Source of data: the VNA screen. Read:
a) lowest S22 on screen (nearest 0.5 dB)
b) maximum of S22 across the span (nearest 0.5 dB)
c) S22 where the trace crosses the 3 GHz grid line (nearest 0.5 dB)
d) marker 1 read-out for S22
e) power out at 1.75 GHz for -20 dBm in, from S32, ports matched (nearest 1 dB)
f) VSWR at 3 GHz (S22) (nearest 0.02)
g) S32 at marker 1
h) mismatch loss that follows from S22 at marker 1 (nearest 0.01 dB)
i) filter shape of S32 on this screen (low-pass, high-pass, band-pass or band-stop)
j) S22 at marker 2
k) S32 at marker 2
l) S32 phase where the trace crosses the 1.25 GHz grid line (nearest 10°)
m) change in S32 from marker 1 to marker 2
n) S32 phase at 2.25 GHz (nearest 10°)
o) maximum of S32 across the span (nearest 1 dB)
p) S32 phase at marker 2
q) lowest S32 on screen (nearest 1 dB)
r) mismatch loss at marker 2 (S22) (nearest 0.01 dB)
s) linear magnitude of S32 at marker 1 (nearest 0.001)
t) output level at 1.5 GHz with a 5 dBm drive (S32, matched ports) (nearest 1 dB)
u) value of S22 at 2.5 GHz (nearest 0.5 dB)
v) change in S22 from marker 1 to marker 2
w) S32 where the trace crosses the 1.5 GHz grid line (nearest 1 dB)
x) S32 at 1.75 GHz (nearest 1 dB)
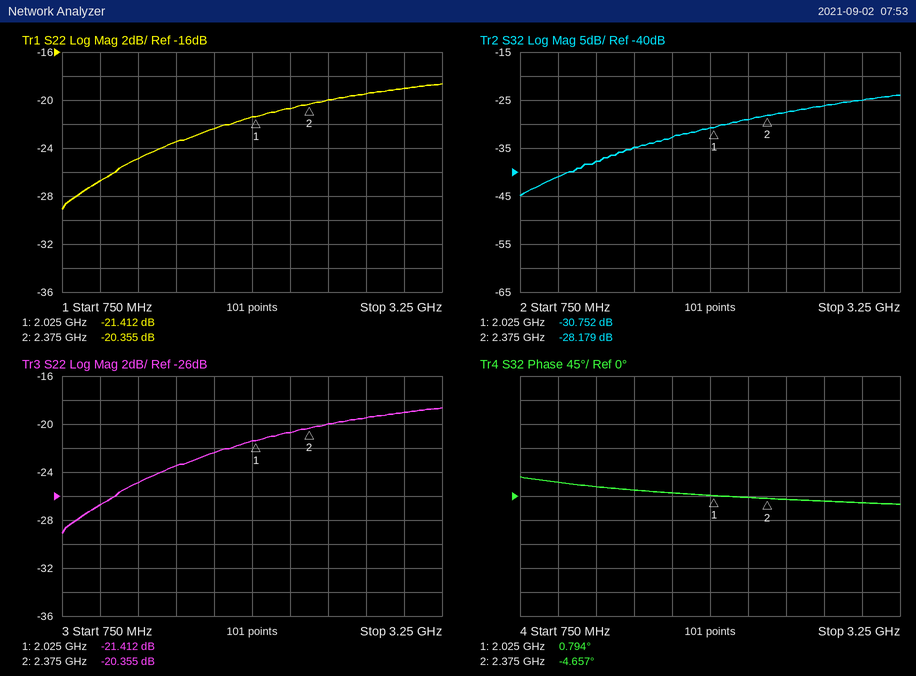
-29.0 dB
-18.5 dB
-19.0 dB
-21.412 dB
-53 dBm
1.26
-30.752 dB
0.03 dB
high-pass
-20.355 dB
-28.179 dB
20°
2.573 dB
0°
-24 dB
-4.657°
-45 dB
0.04 dB
0.029
-30 dBm
-20.0 dB
1.057 dB
-35 dB
-33 dB
